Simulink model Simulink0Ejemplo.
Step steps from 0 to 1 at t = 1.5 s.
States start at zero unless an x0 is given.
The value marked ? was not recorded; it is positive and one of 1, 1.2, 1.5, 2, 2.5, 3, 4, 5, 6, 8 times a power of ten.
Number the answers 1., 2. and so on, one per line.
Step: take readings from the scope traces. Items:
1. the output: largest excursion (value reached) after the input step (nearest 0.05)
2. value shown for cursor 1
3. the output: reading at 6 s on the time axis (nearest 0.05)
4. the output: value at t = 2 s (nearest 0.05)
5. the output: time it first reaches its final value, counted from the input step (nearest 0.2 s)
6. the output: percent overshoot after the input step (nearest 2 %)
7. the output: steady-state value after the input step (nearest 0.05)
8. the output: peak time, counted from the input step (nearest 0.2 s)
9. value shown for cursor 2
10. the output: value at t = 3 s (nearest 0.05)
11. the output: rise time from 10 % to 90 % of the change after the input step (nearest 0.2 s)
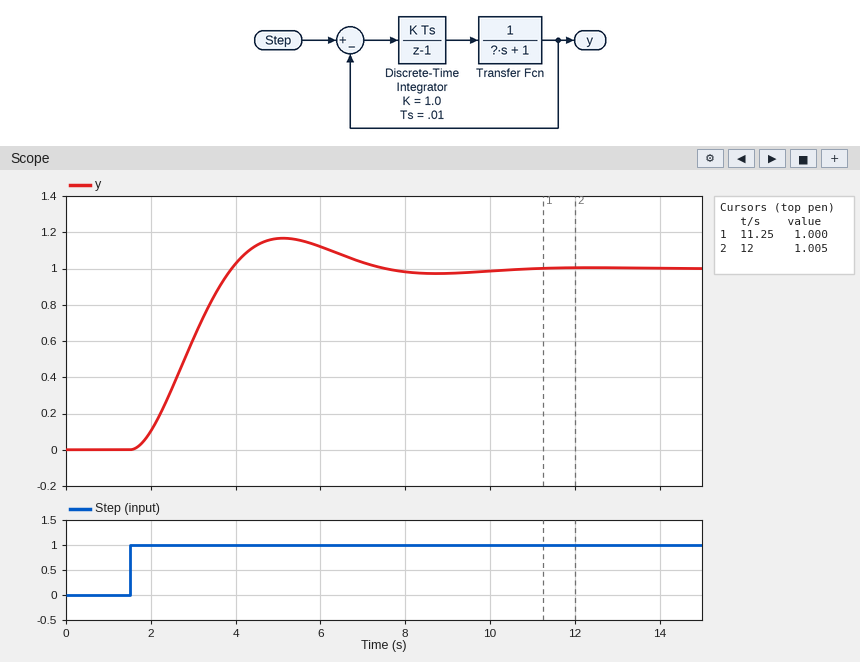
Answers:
1. 1.15
2. 1.000
3. 1.10
4. 0.10
5. 2.4 s
6. 16 %
7. 1.00
8. 3.6 s
9. 1.005
10. 0.60
11. 1.6 s
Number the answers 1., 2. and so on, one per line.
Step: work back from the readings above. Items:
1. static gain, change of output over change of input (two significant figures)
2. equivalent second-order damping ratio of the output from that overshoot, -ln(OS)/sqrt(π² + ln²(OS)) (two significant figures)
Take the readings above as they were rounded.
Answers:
1. 1.0
2. 0.50
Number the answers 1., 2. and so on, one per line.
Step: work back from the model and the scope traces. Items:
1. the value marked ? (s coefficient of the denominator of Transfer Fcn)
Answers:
1. 1
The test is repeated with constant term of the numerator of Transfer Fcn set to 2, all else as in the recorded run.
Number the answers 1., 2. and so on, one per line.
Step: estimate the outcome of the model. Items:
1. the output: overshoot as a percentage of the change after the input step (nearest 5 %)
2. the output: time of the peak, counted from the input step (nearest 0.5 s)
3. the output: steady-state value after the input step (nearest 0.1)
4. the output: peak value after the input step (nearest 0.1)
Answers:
1. 30 %
2. 2.5 s
3. 1.0
4. 1.3
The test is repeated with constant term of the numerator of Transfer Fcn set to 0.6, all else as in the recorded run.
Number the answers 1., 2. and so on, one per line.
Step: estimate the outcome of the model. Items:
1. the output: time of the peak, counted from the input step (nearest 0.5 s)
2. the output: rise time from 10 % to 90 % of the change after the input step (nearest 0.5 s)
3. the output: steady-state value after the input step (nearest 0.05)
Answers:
1. 5.5 s
2. 2.5 s
3. 1.00
